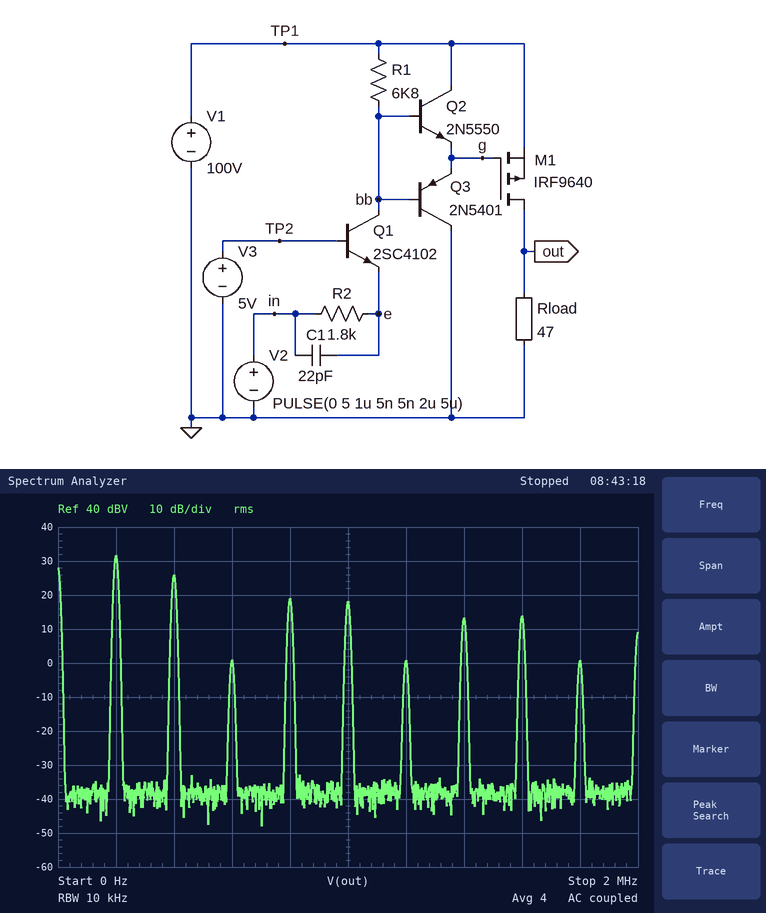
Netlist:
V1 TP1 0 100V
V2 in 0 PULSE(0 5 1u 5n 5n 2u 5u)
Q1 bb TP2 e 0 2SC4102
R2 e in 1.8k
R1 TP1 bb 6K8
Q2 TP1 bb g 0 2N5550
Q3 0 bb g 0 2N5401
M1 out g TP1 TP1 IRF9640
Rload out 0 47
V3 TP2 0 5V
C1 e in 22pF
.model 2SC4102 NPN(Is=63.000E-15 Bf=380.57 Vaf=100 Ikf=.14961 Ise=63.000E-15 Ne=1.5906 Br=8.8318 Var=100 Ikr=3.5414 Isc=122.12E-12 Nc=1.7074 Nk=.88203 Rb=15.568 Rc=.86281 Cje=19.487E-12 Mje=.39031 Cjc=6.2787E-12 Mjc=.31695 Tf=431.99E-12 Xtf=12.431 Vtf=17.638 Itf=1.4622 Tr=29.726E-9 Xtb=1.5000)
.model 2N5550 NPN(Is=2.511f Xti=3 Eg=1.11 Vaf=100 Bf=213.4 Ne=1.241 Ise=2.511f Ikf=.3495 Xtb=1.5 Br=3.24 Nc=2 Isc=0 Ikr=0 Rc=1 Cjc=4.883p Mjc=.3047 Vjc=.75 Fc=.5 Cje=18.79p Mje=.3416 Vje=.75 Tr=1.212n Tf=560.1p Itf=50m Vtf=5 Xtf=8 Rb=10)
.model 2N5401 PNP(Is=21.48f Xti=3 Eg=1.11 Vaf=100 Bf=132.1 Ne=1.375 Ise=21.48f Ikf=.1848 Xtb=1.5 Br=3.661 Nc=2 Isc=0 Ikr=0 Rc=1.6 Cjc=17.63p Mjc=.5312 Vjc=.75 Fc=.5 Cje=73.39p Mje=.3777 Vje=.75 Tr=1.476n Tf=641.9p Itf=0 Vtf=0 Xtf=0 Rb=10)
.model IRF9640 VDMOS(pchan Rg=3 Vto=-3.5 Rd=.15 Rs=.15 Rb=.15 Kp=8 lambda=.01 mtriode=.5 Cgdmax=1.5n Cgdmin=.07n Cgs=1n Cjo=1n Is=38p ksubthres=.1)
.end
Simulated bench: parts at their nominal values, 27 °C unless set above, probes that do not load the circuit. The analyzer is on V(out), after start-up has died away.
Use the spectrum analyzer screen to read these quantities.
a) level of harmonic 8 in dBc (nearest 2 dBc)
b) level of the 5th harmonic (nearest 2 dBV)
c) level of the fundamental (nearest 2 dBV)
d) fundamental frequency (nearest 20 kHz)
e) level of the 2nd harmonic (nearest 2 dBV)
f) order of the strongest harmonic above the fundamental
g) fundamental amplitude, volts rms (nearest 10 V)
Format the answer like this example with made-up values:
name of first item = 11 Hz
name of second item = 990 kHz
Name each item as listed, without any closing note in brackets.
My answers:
level of harmonic 8 in dBc = -18 dBc
level of the 5th harmonic = 18 dBV
level of the fundamental = 32 dBV
fundamental frequency = 200 kHz
level of the 2nd harmonic = 26 dBV
order of the strongest harmonic above the fundamental = 2
fundamental amplitude, volts rms = 40 V
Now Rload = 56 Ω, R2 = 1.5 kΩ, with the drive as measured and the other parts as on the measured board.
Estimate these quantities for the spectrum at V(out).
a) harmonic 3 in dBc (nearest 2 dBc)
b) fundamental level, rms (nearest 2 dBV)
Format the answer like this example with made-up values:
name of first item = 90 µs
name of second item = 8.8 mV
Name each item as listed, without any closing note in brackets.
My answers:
harmonic 3 in dBc = -26 dBc
fundamental level, rms = 32 dBV
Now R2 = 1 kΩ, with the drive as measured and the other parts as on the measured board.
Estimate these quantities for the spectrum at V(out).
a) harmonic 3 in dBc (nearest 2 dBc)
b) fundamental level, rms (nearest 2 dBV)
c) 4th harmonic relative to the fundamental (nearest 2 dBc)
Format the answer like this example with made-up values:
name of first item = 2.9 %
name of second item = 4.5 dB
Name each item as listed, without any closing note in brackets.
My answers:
harmonic 3 in dBc = -20 dBc
fundamental level, rms = 32 dBV
4th harmonic relative to the fundamental = -14 dBc
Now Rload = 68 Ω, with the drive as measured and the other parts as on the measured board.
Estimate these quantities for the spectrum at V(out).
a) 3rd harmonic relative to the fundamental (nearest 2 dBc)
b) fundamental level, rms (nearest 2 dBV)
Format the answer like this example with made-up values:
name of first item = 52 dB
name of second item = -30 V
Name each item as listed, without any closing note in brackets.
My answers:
3rd harmonic relative to the fundamental = -28 dBc
fundamental level, rms = 32 dBV
